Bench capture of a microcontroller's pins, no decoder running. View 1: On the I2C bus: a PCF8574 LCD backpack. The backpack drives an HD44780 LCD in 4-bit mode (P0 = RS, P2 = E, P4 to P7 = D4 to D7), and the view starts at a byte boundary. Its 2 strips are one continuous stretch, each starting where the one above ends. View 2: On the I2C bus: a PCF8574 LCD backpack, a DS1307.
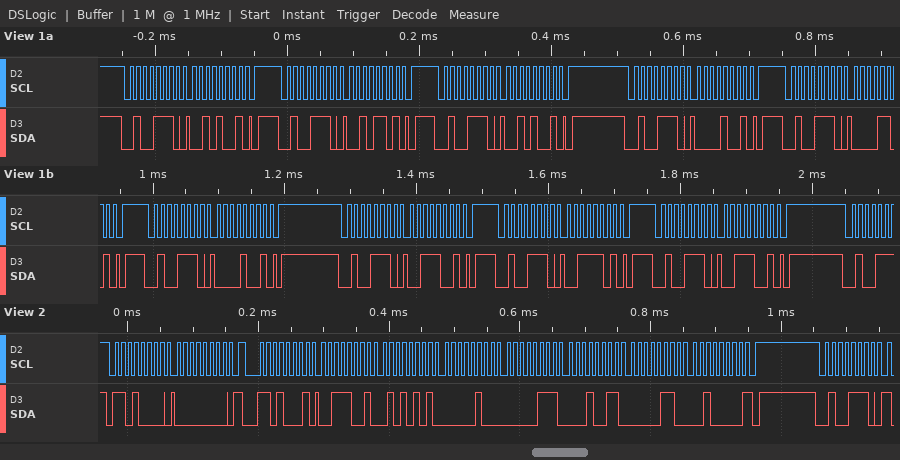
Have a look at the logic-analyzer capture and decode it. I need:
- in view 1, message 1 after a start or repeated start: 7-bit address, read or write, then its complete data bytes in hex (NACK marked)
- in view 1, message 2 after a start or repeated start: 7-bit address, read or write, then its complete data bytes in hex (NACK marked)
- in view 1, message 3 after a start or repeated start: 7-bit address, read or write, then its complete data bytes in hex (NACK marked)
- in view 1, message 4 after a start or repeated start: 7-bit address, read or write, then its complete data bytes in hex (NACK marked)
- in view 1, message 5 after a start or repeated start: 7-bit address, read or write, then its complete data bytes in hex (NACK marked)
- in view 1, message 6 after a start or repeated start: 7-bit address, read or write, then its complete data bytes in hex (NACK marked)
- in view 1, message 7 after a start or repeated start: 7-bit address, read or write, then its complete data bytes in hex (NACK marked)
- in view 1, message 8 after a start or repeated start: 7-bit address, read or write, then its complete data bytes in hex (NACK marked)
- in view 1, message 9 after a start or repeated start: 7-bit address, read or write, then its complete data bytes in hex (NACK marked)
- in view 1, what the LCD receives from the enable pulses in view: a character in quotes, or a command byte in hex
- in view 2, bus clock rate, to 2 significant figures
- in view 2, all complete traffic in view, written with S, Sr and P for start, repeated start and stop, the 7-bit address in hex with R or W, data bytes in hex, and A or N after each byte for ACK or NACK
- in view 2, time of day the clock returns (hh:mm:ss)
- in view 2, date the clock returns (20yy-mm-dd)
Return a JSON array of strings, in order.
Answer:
["0x27 write: 29", "0x27 write: 2D", "0x27 write: 29", "0x27 write: 09", "0x27 write: 0D", "0x27 write: 09", "0x27 write: 39", "0x27 write: 3D", "0x27 write: 39", "' '", "100 kHz", "S 68W A 00 A Sr 68R A 39 A 55 A 04 A 07 A 13 A 06 A 20 N P S 27W A", "04:55:39", "2020-06-13"]
